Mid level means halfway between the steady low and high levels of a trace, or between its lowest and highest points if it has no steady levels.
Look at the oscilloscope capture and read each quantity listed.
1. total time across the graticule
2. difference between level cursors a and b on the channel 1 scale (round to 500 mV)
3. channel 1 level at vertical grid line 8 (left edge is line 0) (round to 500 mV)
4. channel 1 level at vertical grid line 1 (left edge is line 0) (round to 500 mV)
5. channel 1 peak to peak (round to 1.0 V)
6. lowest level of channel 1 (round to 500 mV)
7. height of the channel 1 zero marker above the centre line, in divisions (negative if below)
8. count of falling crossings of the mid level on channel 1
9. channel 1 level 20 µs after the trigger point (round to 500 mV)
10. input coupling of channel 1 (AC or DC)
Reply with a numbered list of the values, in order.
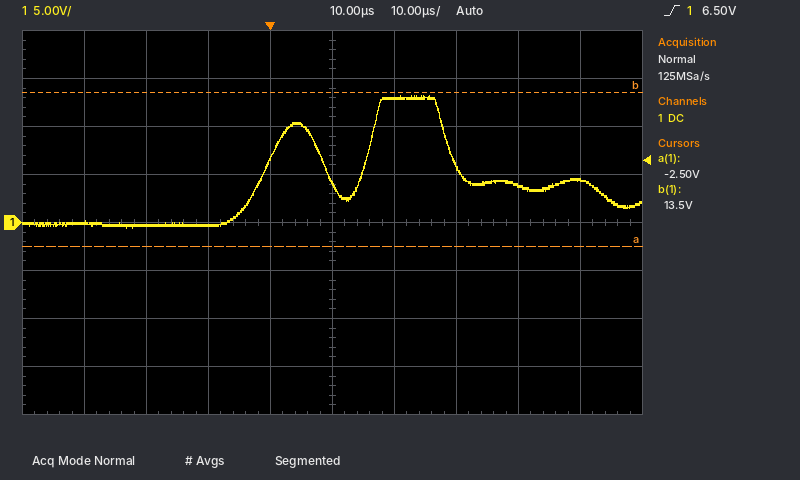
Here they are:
1. 100 µs
2. 16.0 V
3. 4.0 V
4. 0.0 V
5. 14.0 V
6. -500 mV
7. 0.0 div
8. 2
9. 13.0 V
10. DC
